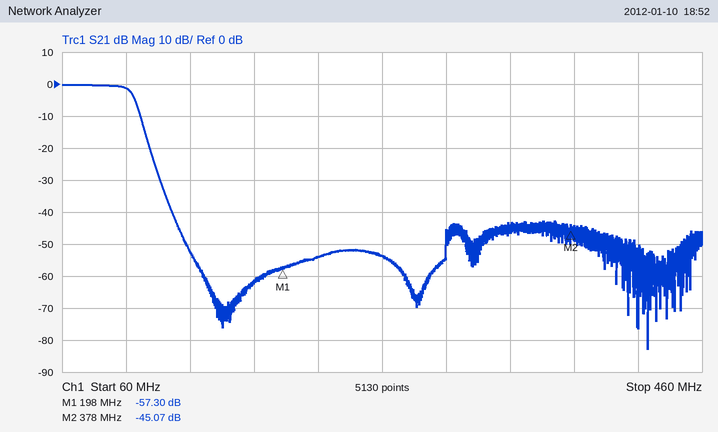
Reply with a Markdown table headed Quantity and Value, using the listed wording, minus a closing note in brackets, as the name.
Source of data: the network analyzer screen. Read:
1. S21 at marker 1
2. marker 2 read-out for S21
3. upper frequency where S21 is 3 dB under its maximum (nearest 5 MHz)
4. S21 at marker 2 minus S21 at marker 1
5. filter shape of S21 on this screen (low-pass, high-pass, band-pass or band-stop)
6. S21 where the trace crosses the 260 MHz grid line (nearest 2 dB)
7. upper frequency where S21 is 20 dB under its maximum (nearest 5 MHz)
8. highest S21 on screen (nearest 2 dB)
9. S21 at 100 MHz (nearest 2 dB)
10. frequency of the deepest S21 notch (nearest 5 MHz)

| Quantity | Value |
|---|---|
| S21 at marker 1 | -57.30 dB |
| marker 2 read-out for S21 | -45.07 dB |
| upper frequency where S21 is 3 dB under its maximum | 105 MHz |
| S21 at marker 2 minus S21 at marker 1 | 12.23 dB |
| filter shape of S21 on this screen | low-pass |
| S21 where the trace crosses the 260 MHz grid line | -54 dB |
| upper frequency where S21 is 20 dB under its maximum | 115 MHz |
| highest S21 on screen | 0 dB |
| S21 at 100 MHz | -2 dB |
| frequency of the deepest S21 notch | 425 MHz |
